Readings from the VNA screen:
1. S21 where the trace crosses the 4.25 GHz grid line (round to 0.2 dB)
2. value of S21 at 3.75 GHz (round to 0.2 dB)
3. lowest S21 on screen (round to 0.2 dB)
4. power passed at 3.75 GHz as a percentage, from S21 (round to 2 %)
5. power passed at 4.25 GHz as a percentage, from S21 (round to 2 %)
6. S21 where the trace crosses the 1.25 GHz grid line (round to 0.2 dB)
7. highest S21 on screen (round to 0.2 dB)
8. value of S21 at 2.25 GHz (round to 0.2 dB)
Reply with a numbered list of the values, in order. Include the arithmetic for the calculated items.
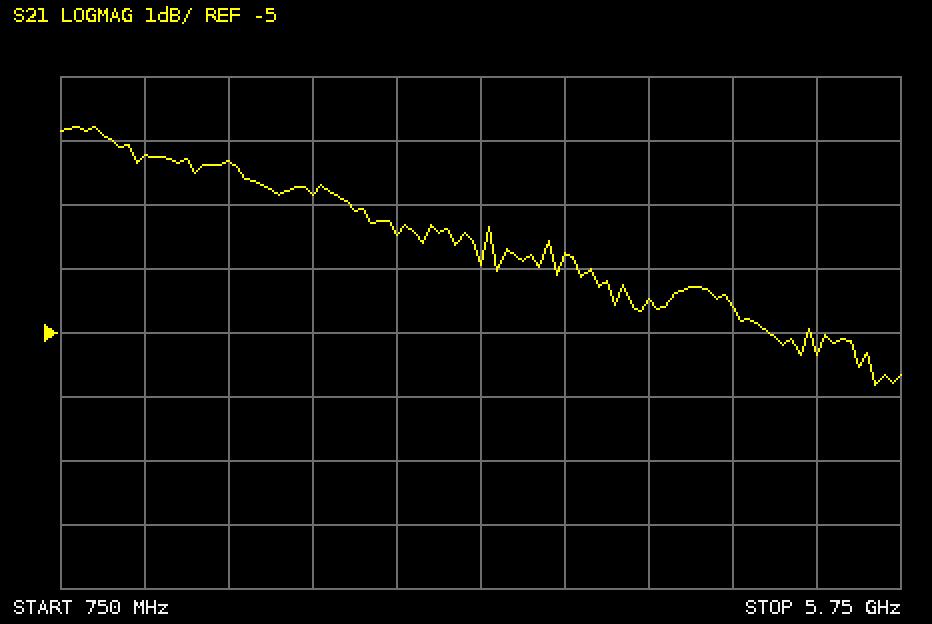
1. -4.4 dB
2. -3.8 dB
3. -5.8 dB
4. 10^(-3.8/10) ≈ 42 %
5. 10^(-4.4/10) ≈ 36 %
6. -2.2 dB
7. -1.8 dB
8. -2.8 dB
